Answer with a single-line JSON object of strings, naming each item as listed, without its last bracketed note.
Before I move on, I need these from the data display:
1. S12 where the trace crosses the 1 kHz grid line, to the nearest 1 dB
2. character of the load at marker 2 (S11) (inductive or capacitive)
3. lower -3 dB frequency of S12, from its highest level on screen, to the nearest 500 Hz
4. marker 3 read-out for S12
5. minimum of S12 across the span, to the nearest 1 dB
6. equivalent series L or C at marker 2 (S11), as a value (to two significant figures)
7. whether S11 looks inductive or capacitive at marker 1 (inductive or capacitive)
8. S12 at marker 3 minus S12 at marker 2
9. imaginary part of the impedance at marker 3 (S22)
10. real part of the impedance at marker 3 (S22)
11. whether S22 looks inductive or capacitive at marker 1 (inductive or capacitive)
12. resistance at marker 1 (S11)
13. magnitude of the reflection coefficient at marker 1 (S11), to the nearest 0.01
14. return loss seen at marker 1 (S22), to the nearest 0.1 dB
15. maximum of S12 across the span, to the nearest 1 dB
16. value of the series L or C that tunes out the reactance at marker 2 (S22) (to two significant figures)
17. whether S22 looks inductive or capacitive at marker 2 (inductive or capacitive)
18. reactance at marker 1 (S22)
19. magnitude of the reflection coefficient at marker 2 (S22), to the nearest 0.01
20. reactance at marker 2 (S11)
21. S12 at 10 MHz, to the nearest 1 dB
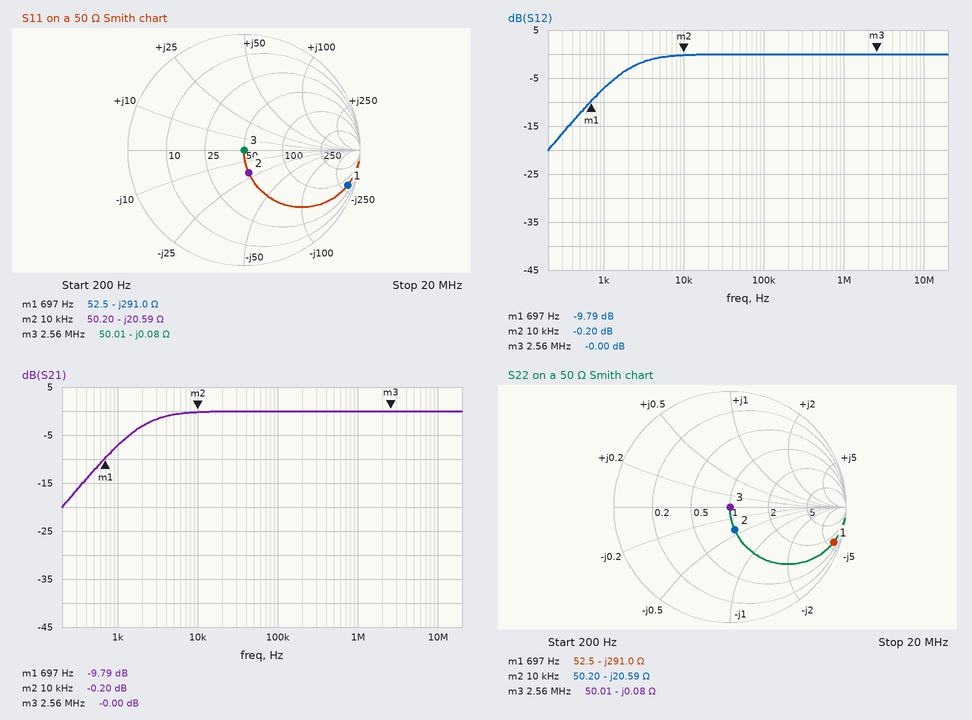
{"S12 where the trace crosses the 1 kHz grid line, to the nearest 1 dB": "-7 dB", "character of the load at marker 2 (S11)": "capacitive", "lower -3 dB frequency of S12, from its highest level on screen, to the nearest 500 Hz": "2.0 kHz", "marker 3 read-out for S12": "-0.00 dB", "minimum of S12 across the span, to the nearest 1 dB": "-20 dB", "equivalent series L or C at marker 2 (S11), as a value": "770 nF", "whether S11 looks inductive or capacitive at marker 1": "capacitive", "S12 at marker 3 minus S12 at marker 2": "0.20 dB", "imaginary part of the impedance at marker 3": "-0.08 Ω", "real part of the impedance at marker 3": "50.01 Ω", "whether S22 looks inductive or capacitive at marker 1": "capacitive", "resistance at marker 1": "52.5 Ω", "magnitude of the reflection coefficient at marker 1 (S11), to the nearest 0.01": "0.94", "return loss seen at marker 1 (S22), to the nearest 0.1 dB": "0.5 dB", "maximum of S12 across the span, to the nearest 1 dB": "0 dB", "value of the series L or C that tunes out the reactance at marker 2 (S22)": "330 µH", "whether S22 looks inductive or capacitive at marker 2": "capacitive", "reactance at marker 1": "-291.0 Ω", "magnitude of the reflection coefficient at marker 2 (S22), to the nearest 0.01": "0.20", "reactance at marker 2": "-20.59 Ω", "S12 at 10 MHz, to the nearest 1 dB": "0 dB"}
